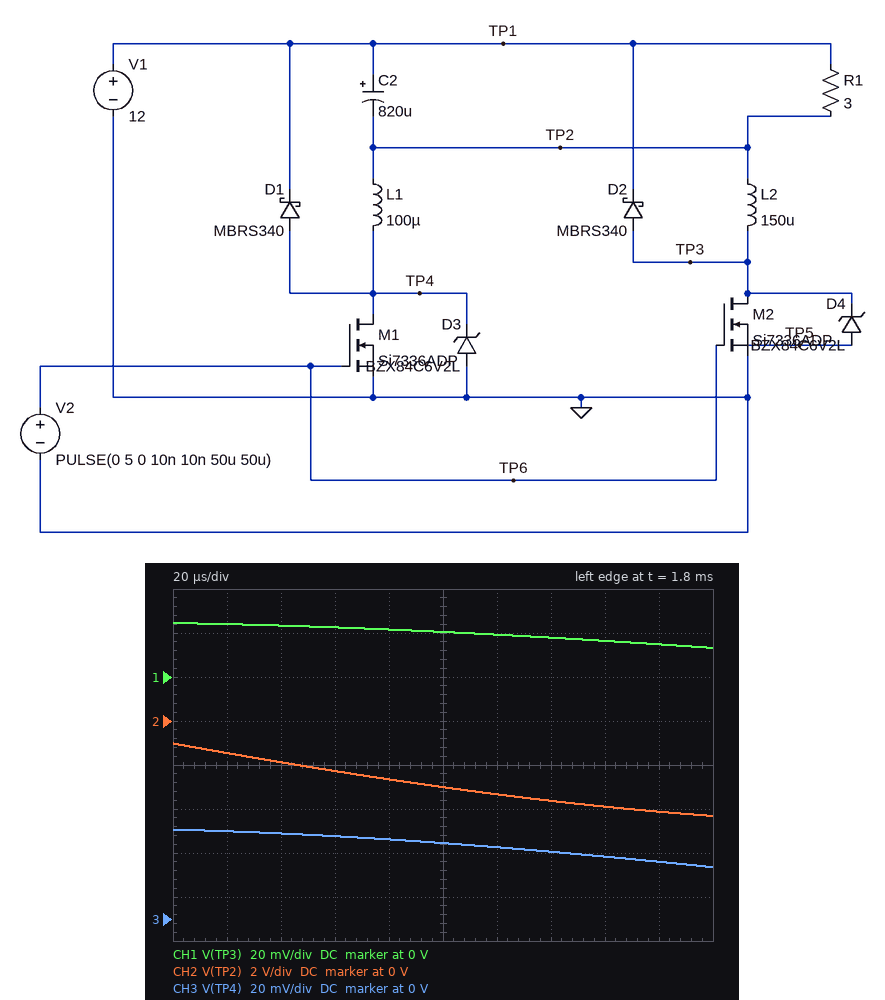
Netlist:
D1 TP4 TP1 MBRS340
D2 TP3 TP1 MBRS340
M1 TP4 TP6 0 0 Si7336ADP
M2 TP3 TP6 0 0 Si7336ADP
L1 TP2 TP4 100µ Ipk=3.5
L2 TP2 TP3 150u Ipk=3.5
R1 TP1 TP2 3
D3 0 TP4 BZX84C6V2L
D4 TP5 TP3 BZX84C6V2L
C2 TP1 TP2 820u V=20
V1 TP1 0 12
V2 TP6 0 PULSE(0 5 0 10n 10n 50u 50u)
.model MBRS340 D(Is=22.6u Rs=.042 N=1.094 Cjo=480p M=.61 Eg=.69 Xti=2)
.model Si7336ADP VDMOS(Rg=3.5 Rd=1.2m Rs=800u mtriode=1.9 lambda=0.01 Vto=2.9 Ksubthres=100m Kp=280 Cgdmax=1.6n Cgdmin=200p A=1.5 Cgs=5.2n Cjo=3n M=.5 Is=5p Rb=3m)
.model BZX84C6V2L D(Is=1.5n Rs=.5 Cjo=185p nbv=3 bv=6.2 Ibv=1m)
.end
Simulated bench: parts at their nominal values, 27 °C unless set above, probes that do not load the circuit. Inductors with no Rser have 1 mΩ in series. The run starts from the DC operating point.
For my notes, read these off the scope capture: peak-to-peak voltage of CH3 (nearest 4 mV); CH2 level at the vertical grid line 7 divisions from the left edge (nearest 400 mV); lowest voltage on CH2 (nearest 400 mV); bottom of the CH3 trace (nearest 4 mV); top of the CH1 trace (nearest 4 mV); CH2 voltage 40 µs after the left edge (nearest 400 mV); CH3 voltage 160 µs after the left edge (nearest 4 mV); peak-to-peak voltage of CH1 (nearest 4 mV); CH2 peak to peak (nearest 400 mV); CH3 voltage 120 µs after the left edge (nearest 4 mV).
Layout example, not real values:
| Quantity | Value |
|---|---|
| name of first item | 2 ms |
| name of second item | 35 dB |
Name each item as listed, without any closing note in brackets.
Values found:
| Quantity | Value |
|---|---|
| peak-to-peak voltage of CH3 | 16 mV |
| CH2 level at the vertical grid line 7 divisions from the left edge | -3.6 V |
| lowest voltage on CH2 | -4.4 V |
| bottom of the CH3 trace | 24 mV |
| top of the CH1 trace | 24 mV |
| CH2 voltage 40 µs after the left edge | -2.0 V |
| CH3 voltage 160 µs after the left edge | 28 mV |
| peak-to-peak voltage of CH1 | 12 mV |
| CH2 peak to peak | 3.2 V |
| CH3 voltage 120 µs after the left edge | 32 mV |
